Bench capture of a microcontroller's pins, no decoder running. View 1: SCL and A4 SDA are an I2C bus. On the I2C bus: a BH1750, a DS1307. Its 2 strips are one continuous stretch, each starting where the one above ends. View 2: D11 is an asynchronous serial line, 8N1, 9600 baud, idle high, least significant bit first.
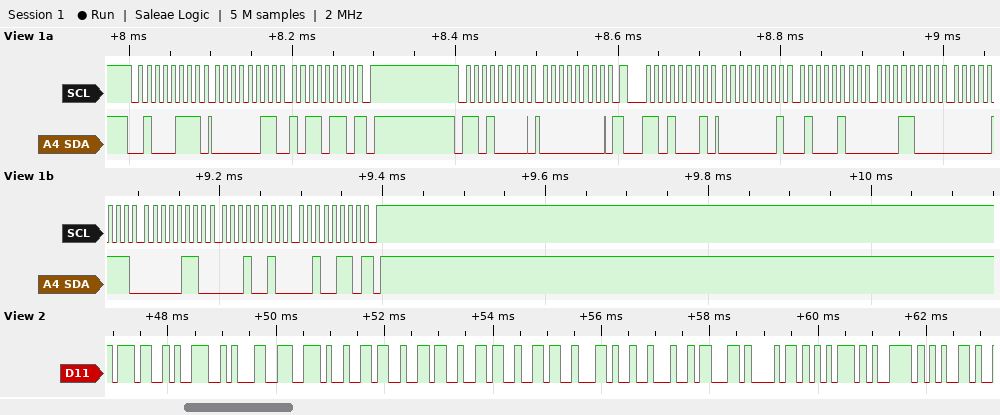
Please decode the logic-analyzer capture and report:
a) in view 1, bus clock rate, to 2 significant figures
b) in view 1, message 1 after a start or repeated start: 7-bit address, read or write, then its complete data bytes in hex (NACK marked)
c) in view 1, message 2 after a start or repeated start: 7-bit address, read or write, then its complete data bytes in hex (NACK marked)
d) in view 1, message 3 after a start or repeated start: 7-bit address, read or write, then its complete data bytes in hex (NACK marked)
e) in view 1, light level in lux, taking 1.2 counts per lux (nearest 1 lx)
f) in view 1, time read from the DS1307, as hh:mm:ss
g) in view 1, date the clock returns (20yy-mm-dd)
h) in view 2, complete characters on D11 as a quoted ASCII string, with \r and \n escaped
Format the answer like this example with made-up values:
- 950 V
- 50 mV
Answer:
- 100 kHz
- 0x23 read: 03 B6 NACK
- 0x68 write: 00
- 0x68 read: 01 44 18 07 06 12 26 NACK
- 792 lx
- 18:44:01
- 2026-12-06
- "791.6666,\"chuye"
